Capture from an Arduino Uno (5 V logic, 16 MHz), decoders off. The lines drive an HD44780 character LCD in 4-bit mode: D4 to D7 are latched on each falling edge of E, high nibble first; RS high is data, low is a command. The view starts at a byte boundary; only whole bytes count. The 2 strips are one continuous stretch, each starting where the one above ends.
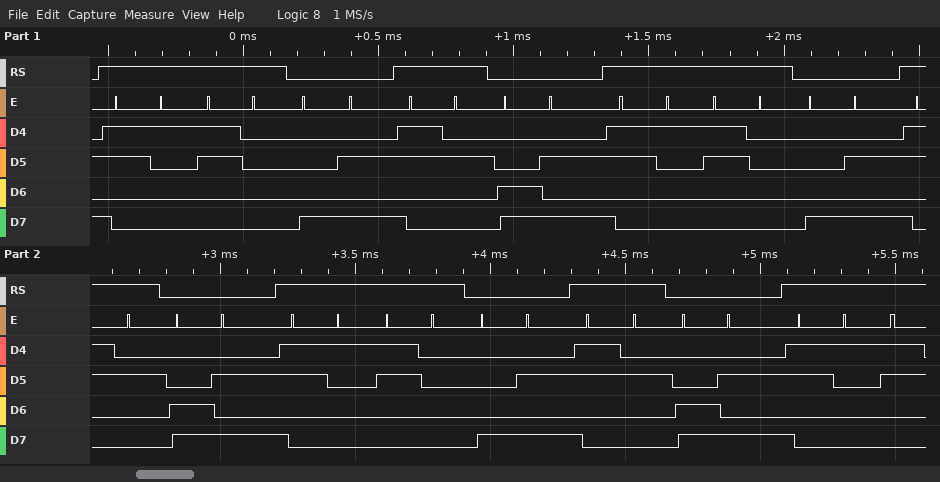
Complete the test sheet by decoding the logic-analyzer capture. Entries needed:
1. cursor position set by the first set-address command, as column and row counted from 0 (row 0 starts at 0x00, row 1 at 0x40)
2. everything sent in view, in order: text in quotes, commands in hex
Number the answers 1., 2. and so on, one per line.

1. column 10, row 0
2. "10" 0x8A "2" 0xCA "10" 0x8A "2" 0xCA "10" 0x8A "2" 0xCA "1"
